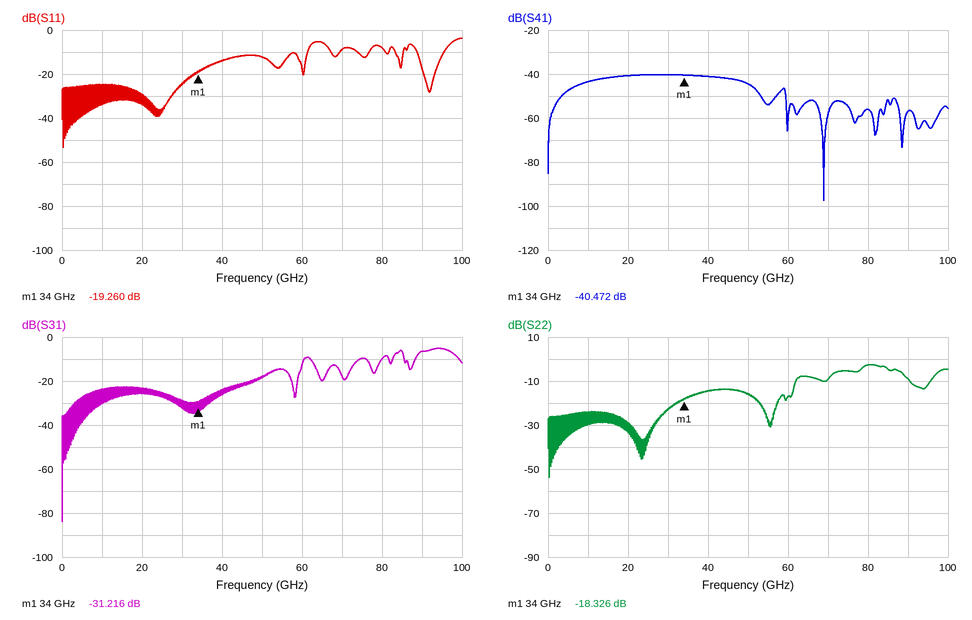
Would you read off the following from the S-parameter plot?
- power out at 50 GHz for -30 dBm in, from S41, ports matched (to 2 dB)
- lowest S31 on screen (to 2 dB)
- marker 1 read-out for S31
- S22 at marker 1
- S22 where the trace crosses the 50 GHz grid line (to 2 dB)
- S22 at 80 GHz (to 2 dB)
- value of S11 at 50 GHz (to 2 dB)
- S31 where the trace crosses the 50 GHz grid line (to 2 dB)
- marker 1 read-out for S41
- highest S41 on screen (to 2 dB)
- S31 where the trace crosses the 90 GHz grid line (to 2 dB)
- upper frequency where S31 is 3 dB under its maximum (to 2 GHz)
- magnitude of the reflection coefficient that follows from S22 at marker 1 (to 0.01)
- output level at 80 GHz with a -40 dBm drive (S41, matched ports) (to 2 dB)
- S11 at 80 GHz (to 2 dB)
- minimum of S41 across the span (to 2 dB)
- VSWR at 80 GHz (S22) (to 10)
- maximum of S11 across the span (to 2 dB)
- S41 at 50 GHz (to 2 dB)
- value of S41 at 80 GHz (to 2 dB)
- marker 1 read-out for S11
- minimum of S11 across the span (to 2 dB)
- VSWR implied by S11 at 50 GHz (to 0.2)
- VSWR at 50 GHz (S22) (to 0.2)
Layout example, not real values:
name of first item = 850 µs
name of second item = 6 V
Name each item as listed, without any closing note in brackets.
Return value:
power out at 50 GHz for -30 dBm in, from S41, ports matched = -74 dBm
lowest S31 on screen = -84 dB
marker 1 read-out for S31 = -31.216 dB
S22 at marker 1 = -18.326 dB
S22 where the trace crosses the 50 GHz grid line = -16 dB
S22 at 80 GHz = -2 dB
value of S11 at 50 GHz = -12 dB
S31 where the trace crosses the 50 GHz grid line = -18 dB
marker 1 read-out for S41 = -40.472 dB
highest S41 on screen = -40 dB
S31 where the trace crosses the 90 GHz grid line = -6 dB
upper frequency where S31 is 3 dB under its maximum = 98 GHz
magnitude of the reflection coefficient that follows from S22 at marker 1 = 0.12
output level at 80 GHz with a -40 dBm drive (S41, matched ports) = -96 dBm
S11 at 80 GHz = -8 dB
minimum of S41 across the span = -98 dB
VSWR at 80 GHz (S22) = 10
maximum of S11 across the span = -4 dB
S41 at 50 GHz = -44 dB
value of S41 at 80 GHz = -56 dB
marker 1 read-out for S11 = -19.260 dB
minimum of S11 across the span = -54 dB
VSWR implied by S11 at 50 GHz = 1.6
VSWR at 50 GHz (S22) = 1.4
